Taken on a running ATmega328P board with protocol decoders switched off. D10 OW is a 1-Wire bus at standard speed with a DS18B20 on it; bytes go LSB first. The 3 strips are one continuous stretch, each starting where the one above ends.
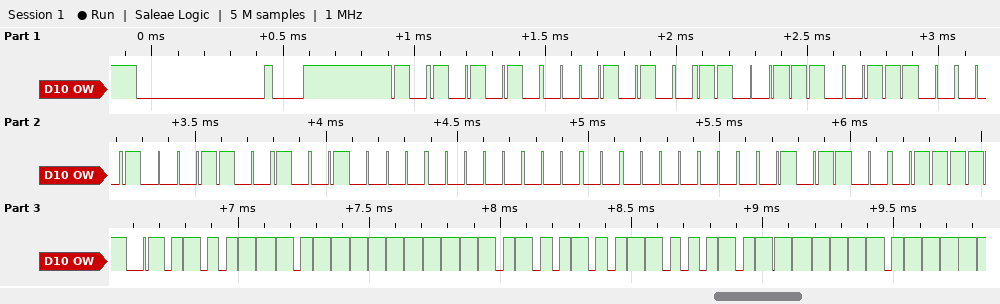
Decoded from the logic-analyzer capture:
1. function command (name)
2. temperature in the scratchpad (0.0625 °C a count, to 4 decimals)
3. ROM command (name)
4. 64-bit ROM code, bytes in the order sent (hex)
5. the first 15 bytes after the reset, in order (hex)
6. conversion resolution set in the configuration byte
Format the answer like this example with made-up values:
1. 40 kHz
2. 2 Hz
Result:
1. Read Scratchpad
2. -8.8750 °C
3. Match ROM
4. 28 73 0E 31 09 00 00 34
5. 55 28 73 0E 31 09 00 00 34 BE 72 FF 4B 46 7F
6. 12 bits
